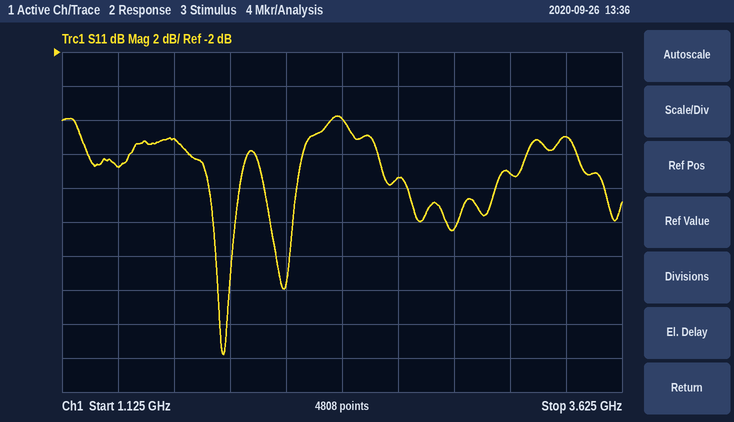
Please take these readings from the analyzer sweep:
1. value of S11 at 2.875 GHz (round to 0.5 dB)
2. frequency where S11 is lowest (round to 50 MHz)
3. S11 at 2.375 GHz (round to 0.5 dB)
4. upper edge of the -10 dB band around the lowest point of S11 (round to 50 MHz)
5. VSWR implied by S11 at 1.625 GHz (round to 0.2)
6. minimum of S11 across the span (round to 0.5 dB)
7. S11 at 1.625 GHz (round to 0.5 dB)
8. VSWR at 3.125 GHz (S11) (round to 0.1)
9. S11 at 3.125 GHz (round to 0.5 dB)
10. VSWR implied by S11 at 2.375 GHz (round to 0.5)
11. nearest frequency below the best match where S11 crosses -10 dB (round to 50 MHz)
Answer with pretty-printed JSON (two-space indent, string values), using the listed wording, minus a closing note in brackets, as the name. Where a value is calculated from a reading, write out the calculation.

{
  "value of S11 at 2.875 GHz": "-12.5 dB",
  "frequency where S11 is lowest": "1.85 GHz",
  "S11 at 2.375 GHz": "-6.0 dB",
  "upper edge of the -10 dB band around the lowest point of S11": "1.90 GHz",
  "VSWR implied by S11 at 1.625 GHz": "|Γ| = 10^(-7/20) = 0.4467; VSWR = (1 + 0.4467)/(1 − 0.4467) ≈ 2.6",
  "minimum of S11 across the span": "-20.0 dB",
  "S11 at 1.625 GHz": "-7.0 dB",
  "VSWR at 3.125 GHz (S11)": "|Γ| = 10^(-9/20) = 0.3548; VSWR = (1 + 0.3548)/(1 − 0.3548) ≈ 2.1",
  "S11 at 3.125 GHz": "-9.0 dB",
  "VSWR implied by S11 at 2.375 GHz": "|Γ| = 10^(-6/20) = 0.5012; VSWR = (1 + 0.5012)/(1 − 0.5012) ≈ 3.0",
  "nearest frequency below the best match where S11 crosses -10 dB": "1.80 GHz"
}
